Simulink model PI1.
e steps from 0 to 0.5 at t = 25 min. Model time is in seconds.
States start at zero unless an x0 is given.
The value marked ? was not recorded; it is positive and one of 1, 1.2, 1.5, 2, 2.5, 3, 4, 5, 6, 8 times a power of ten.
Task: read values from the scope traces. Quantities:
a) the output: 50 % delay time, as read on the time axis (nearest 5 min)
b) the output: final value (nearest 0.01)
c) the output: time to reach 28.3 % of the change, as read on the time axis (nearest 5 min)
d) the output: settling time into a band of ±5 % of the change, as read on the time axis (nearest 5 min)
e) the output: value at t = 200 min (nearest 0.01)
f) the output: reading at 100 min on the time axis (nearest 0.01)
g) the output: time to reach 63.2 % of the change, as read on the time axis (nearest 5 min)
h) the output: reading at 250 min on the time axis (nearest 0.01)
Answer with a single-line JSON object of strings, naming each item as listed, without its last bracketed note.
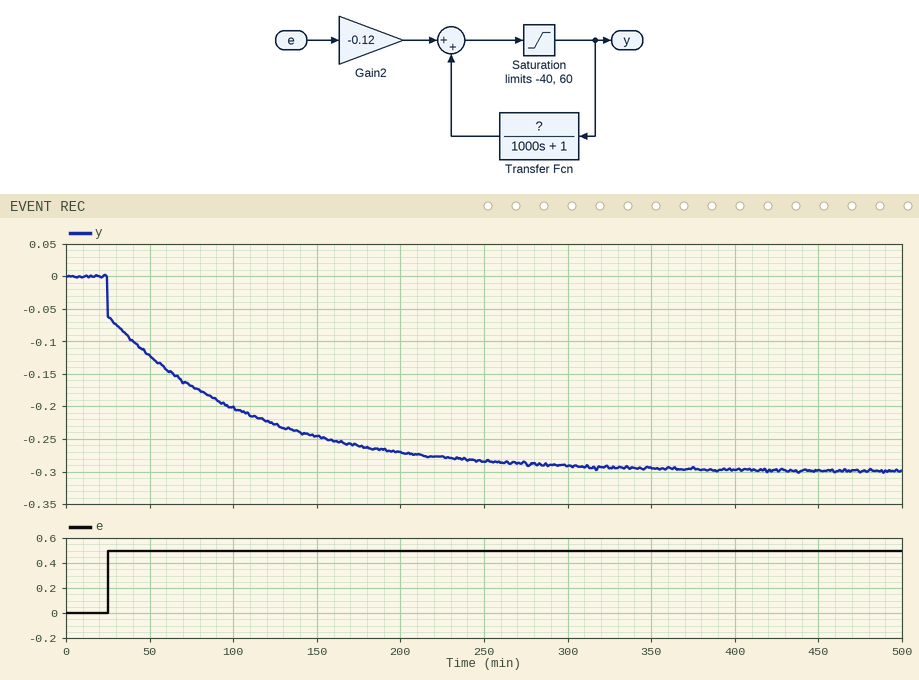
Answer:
{"the output: 50 % delay time, as read on the time axis": "65 min", "the output: final value": "-0.30", "the output: time to reach 28.3 % of the change, as read on the time axis": "35 min", "the output: settling time into a band of ±5 % of the change, as read on the time axis": "255 min", "the output: value at t = 200 min": "-0.27", "the output: reading at 100 min on the time axis": "-0.20", "the output: time to reach 63.2 % of the change, as read on the time axis": "90 min", "the output: reading at 250 min on the time axis": "-0.28"}
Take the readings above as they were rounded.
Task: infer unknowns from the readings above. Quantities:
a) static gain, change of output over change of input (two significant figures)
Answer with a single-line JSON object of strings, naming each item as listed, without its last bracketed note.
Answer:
{"static gain, change of output over change of input": "-0.60"}
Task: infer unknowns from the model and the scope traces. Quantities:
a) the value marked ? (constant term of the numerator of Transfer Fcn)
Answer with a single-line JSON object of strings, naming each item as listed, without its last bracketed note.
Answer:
{"the value marked ?": "0.8"}
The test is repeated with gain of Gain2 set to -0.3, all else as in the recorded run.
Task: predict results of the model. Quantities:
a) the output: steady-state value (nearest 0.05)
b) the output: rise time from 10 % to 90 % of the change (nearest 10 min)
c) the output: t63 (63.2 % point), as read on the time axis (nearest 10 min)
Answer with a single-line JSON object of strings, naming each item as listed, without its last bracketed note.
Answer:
{"the output: steady-state value": "-0.75", "the output: rise time from 10 % to 90 % of the change": "170 min", "the output: t63 (63.2 % point), as read on the time axis": "90 min"}
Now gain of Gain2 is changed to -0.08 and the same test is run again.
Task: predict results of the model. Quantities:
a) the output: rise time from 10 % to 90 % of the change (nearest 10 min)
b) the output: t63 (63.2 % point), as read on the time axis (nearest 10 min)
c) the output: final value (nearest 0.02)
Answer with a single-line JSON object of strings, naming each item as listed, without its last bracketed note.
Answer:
{"the output: rise time from 10 % to 90 % of the change": "170 min", "the output: t63 (63.2 % point), as read on the time axis": "90 min", "the output: final value": "-0.20"}
